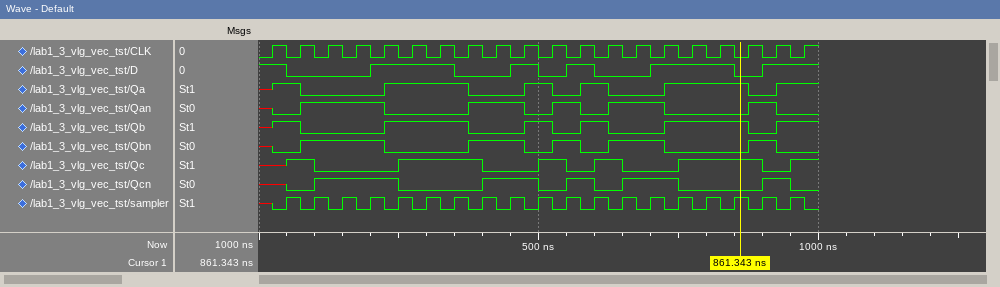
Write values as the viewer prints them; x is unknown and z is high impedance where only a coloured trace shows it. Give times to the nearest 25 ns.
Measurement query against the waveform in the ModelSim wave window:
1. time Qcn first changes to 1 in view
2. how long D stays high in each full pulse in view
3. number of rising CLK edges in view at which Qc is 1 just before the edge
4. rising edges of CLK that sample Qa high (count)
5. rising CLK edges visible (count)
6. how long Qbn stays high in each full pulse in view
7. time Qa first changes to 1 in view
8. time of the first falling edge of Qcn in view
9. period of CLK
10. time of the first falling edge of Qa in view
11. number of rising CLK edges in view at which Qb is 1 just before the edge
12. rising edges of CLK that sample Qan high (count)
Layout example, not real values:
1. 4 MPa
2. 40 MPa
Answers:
1. 100 ns
2. 150 ns, 50 ns, 50 ns, 150 ns
3. 10
4. 10
5. 20
6. 150 ns, 100 ns, 50 ns, 100 ns, 50 ns
7. 25 ns
8. 250 ns
9. 50 ns
10. 75 ns
11. 10
12. 9
